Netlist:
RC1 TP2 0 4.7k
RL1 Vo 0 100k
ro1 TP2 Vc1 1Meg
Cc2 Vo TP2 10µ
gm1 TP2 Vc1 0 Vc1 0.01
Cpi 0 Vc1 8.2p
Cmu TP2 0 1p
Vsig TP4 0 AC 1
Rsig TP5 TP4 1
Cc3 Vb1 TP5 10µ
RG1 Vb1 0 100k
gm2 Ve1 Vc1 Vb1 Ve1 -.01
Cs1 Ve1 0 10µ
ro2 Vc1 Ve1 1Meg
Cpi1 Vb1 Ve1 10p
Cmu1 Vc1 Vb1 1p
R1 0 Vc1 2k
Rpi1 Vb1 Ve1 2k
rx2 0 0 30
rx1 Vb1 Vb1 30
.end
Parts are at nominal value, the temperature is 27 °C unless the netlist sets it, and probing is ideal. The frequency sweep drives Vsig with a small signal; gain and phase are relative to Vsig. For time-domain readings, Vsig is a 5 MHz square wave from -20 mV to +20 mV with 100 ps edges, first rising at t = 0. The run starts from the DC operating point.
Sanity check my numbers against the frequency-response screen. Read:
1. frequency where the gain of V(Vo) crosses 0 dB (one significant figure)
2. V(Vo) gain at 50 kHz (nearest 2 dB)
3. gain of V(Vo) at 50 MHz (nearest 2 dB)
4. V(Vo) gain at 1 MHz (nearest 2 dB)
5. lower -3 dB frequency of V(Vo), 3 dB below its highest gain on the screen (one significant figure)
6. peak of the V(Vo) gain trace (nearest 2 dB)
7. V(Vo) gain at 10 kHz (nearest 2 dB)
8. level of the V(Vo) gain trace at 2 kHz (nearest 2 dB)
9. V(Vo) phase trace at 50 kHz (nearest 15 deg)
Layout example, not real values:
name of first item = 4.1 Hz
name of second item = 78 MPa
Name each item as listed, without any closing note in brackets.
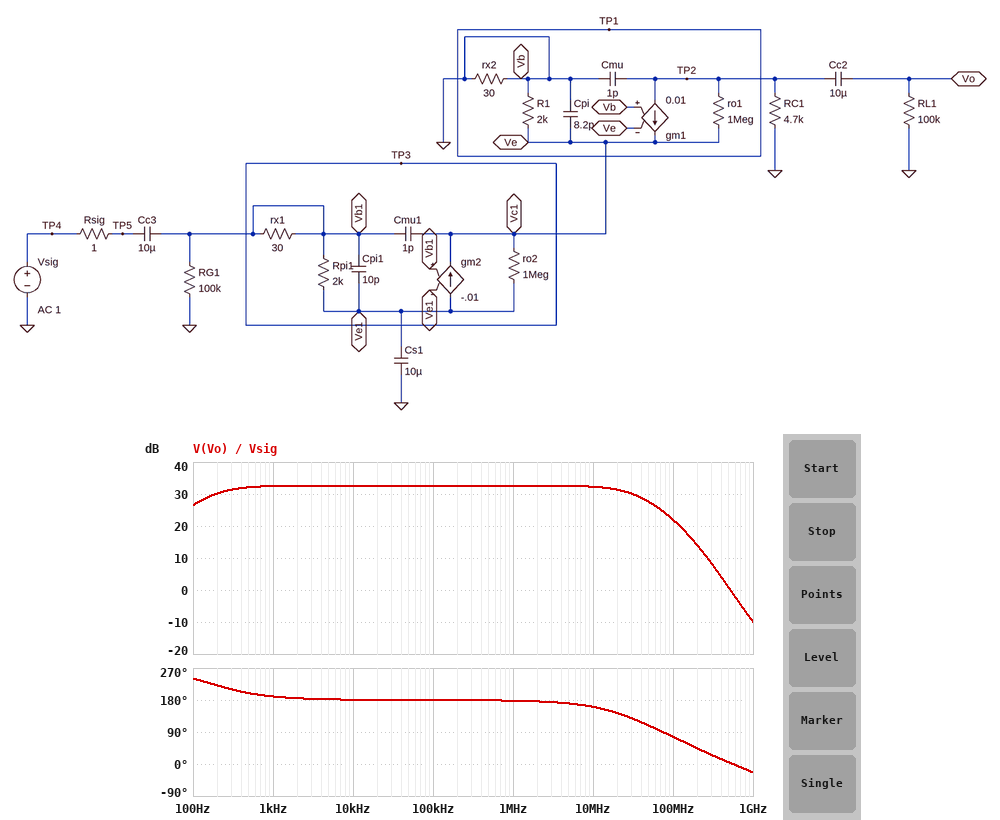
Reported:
frequency where the gain of V(Vo) crosses 0 dB = 500 MHz
V(Vo) gain at 50 kHz = 32 dB
gain of V(Vo) at 50 MHz = 28 dB
V(Vo) gain at 1 MHz = 32 dB
lower -3 dB frequency of V(Vo), 3 dB below its highest gain on the screen = 200 Hz
peak of the V(Vo) gain trace = 32 dB
V(Vo) gain at 10 kHz = 32 dB
level of the V(Vo) gain trace at 2 kHz = 32 dB
V(Vo) phase trace at 50 kHz = 180 deg
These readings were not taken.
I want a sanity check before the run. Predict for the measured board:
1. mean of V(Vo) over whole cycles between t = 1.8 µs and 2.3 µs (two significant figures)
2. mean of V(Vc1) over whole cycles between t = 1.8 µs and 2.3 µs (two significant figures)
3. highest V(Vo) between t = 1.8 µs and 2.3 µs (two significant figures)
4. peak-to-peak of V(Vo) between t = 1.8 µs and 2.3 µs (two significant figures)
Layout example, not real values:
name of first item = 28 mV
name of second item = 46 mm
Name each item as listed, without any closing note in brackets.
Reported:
mean of V(Vo) over whole cycles between t = 1.8 µs and 2.3 µs = -850 mV
mean of V(Vc1) over whole cycles between t = 1.8 µs and 2.3 µs = -19 mV
highest V(Vo) between t = 1.8 µs and 2.3 µs = 3.8 mV
peak-to-peak of V(Vo) between t = 1.8 µs and 2.3 µs = 1.7 V
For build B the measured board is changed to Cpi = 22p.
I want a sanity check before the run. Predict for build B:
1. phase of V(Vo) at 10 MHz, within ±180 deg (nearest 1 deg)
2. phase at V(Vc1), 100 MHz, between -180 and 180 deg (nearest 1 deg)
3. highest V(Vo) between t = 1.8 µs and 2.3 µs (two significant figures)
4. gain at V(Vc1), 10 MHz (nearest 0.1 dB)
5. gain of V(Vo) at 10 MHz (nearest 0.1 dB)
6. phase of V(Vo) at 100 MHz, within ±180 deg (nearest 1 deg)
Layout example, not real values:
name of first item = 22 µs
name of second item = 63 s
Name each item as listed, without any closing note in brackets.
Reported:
phase of V(Vo) at 10 MHz, within ±180 deg = 156 deg
phase at V(Vc1), 100 MHz, between -180 and 180 deg = 122 deg
highest V(Vo) between t = 1.8 µs and 2.3 µs = 2.8 mV
gain at V(Vc1), 10 MHz = -0.5 dB
gain of V(Vo) at 10 MHz = 32.2 dB
phase of V(Vo) at 100 MHz, within ±180 deg = 52 deg
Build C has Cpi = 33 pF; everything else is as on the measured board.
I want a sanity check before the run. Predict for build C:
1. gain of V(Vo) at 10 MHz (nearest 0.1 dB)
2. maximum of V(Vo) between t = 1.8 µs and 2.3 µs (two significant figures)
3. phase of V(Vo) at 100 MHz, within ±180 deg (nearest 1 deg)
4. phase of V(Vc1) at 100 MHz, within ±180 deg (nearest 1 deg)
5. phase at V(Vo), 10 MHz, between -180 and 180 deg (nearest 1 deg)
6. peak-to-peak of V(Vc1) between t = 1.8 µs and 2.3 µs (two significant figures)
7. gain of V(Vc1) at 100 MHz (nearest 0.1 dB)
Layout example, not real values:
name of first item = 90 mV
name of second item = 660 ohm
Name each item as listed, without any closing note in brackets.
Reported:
gain of V(Vo) at 10 MHz = 32.1 dB
maximum of V(Vo) between t = 1.8 µs and 2.3 µs = 2.6 mV
phase of V(Vo) at 100 MHz, within ±180 deg = 42 deg
phase of V(Vc1) at 100 MHz, within ±180 deg = 112 deg
phase at V(Vo), 10 MHz, between -180 and 180 deg = 152 deg
peak-to-peak of V(Vc1) between t = 1.8 µs and 2.3 µs = 39 mV
gain of V(Vc1) at 100 MHz = -7.5 dB
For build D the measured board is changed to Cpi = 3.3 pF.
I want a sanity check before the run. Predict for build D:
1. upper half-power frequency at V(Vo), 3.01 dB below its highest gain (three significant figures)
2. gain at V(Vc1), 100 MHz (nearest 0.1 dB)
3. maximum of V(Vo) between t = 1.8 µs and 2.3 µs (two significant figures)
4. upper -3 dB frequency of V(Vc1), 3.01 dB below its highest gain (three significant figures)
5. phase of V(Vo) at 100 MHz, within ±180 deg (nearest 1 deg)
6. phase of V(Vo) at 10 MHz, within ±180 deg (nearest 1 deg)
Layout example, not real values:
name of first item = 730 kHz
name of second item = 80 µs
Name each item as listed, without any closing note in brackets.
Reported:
upper half-power frequency at V(Vo), 3.01 dB below its highest gain = 35.2 MHz
gain at V(Vc1), 100 MHz = -0.7 dB
maximum of V(Vo) between t = 1.8 µs and 2.3 µs = 5.5 mV
upper -3 dB frequency of V(Vc1), 3.01 dB below its highest gain = 409 MHz
phase of V(Vo) at 100 MHz, within ±180 deg = 91 deg
phase of V(Vo) at 10 MHz, within ±180 deg = 162 deg
